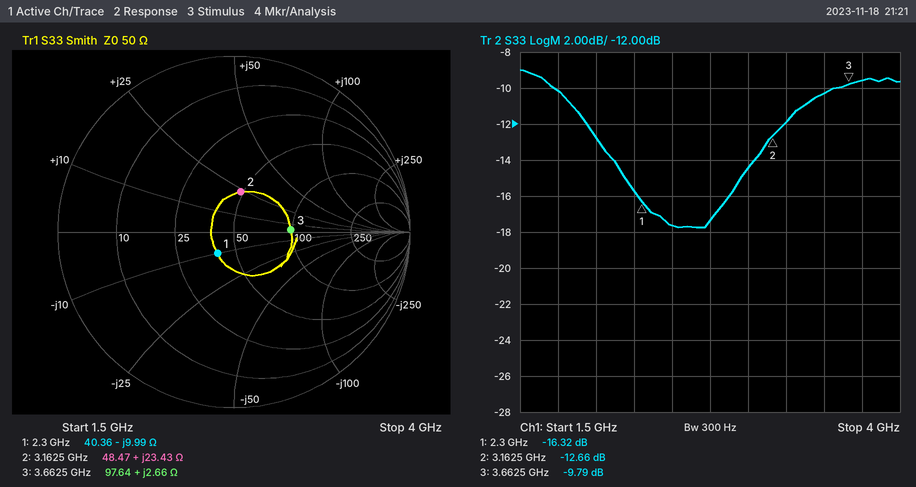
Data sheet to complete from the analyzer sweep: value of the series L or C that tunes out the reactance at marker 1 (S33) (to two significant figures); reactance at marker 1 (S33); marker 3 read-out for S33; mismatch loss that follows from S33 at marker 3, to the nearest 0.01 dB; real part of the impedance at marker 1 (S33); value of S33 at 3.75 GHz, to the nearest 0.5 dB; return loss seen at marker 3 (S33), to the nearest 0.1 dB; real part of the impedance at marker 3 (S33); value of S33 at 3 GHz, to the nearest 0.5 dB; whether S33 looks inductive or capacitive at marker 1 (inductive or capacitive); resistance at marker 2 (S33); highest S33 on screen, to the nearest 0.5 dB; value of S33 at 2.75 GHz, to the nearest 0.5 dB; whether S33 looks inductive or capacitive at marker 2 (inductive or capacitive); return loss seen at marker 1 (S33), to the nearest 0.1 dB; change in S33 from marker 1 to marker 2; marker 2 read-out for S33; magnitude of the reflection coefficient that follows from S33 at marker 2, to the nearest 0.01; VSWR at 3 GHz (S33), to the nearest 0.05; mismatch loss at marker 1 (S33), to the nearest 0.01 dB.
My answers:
690 pH
-9.99 Ω
-9.79 dB
0.48 dB
40.36 Ω
-9.5 dB
9.8 dB
97.64 Ω
-14.5 dB
capacitive
48.47 Ω
-9.0 dB
-17.5 dB
inductive
16.3 dB
3.66 dB
-12.66 dB
0.23
1.45
0.10 dB
